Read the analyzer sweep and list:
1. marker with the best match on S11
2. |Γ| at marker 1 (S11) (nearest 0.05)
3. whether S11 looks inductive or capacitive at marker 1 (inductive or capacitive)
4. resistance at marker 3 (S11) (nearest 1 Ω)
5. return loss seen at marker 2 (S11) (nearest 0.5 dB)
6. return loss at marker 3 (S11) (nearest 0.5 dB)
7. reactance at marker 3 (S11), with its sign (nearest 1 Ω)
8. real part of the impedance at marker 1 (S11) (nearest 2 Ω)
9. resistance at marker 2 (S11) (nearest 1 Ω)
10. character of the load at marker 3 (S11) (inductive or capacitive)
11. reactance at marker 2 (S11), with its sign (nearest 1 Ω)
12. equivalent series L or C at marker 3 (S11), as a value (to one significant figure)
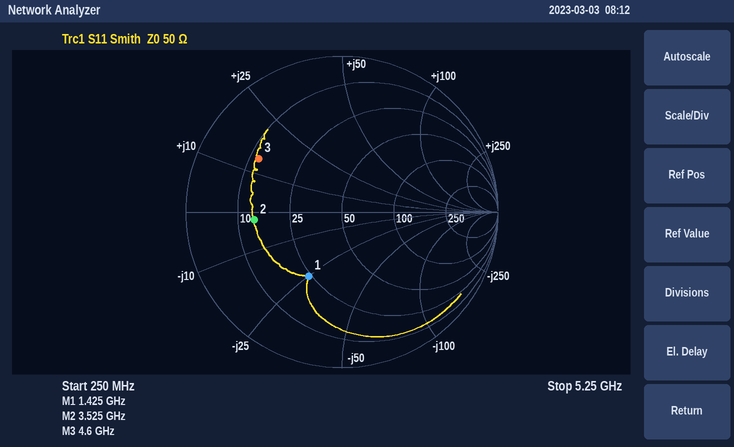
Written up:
marker 1
0.45
capacitive
12 Ω
5.0 dB
4.0 dB
+14 Ω
24 Ω
14 Ω
inductive
-2 Ω
500 pH
